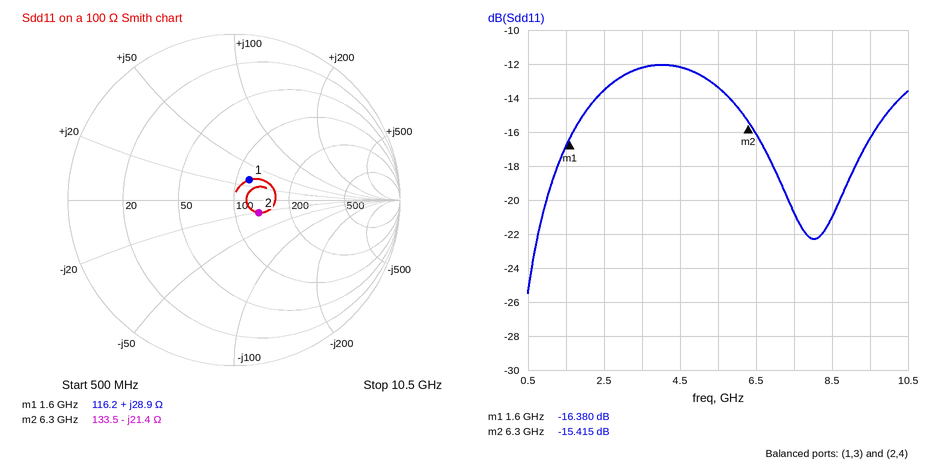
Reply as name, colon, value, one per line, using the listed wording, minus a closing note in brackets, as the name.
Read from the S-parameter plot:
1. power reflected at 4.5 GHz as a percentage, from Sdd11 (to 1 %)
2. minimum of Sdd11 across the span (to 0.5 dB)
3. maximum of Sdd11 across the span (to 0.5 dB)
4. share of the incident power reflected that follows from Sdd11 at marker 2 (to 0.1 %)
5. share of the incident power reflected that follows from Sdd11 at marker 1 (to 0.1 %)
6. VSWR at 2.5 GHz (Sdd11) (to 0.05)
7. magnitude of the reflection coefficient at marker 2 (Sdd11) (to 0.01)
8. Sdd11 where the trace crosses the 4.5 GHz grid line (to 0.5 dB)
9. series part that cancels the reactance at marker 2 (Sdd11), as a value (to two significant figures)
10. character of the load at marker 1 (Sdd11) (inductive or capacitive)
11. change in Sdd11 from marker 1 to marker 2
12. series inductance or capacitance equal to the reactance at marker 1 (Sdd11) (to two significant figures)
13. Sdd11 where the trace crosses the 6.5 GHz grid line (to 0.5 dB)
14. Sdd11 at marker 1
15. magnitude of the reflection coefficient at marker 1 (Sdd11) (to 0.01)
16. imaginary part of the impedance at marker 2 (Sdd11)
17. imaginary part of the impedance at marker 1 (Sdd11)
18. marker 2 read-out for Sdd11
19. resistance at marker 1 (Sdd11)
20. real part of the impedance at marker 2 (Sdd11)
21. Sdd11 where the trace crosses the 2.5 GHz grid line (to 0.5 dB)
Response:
power reflected at 4.5 GHz as a percentage, from Sdd11: 6 %
minimum of Sdd11 across the span: -25.5 dB
maximum of Sdd11 across the span: -12.0 dB
share of the incident power reflected that follows from Sdd11 at marker 2: 2.9 %
share of the incident power reflected that follows from Sdd11 at marker 1: 2.3 %
VSWR at 2.5 GHz (Sdd11): 1.55
magnitude of the reflection coefficient at marker 2 (Sdd11): 0.17
Sdd11 where the trace crosses the 4.5 GHz grid line: -12.0 dB
series part that cancels the reactance at marker 2 (Sdd11), as a value: 540 pH
character of the load at marker 1 (Sdd11): inductive
change in Sdd11 from marker 1 to marker 2: 0.965 dB
series inductance or capacitance equal to the reactance at marker 1 (Sdd11): 2.9 nH
Sdd11 where the trace crosses the 6.5 GHz grid line: -16.0 dB
Sdd11 at marker 1: -16.380 dB
magnitude of the reflection coefficient at marker 1 (Sdd11): 0.15
imaginary part of the impedance at marker 2: -21.4 Ω
imaginary part of the impedance at marker 1: +28.9 Ω
marker 2 read-out for Sdd11: -15.415 dB
resistance at marker 1: 116.2 Ω
real part of the impedance at marker 2: 133.5 Ω
Sdd11 where the trace crosses the 2.5 GHz grid line: -13.5 dB
